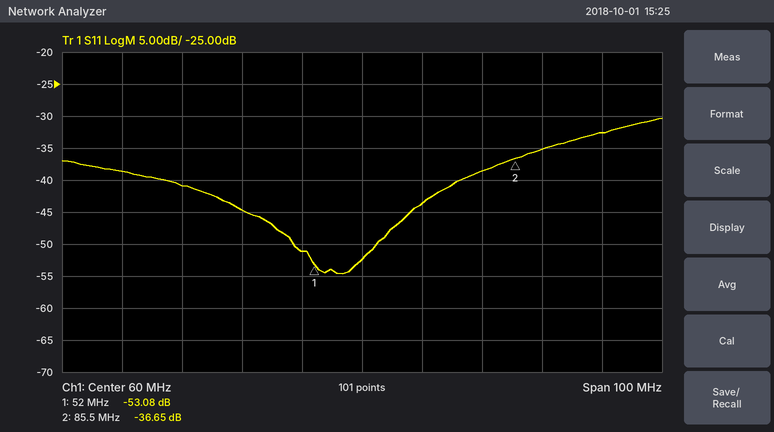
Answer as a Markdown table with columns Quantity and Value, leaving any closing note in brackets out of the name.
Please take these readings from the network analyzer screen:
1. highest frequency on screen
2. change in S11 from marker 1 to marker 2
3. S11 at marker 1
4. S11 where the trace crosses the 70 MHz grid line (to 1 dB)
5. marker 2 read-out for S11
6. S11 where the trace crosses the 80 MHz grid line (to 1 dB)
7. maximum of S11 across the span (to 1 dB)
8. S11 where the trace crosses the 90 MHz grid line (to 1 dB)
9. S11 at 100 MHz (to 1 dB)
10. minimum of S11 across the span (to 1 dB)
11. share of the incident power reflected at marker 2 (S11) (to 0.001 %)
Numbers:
| Quantity | Value |
|---|---|
| highest frequency on screen | 110 MHz |
| change in S11 from marker 1 to marker 2 | 16.43 dB |
| S11 at marker 1 | -53.08 dB |
| S11 where the trace crosses the 70 MHz grid line | -44 dB |
| marker 2 read-out for S11 | -36.65 dB |
| S11 where the trace crosses the 80 MHz grid line | -39 dB |
| maximum of S11 across the span | -30 dB |
| S11 where the trace crosses the 90 MHz grid line | -35 dB |
| S11 at 100 MHz | -33 dB |
| minimum of S11 across the span | -55 dB |
| share of the incident power reflected at marker 2 (S11) | 0.022 % |
